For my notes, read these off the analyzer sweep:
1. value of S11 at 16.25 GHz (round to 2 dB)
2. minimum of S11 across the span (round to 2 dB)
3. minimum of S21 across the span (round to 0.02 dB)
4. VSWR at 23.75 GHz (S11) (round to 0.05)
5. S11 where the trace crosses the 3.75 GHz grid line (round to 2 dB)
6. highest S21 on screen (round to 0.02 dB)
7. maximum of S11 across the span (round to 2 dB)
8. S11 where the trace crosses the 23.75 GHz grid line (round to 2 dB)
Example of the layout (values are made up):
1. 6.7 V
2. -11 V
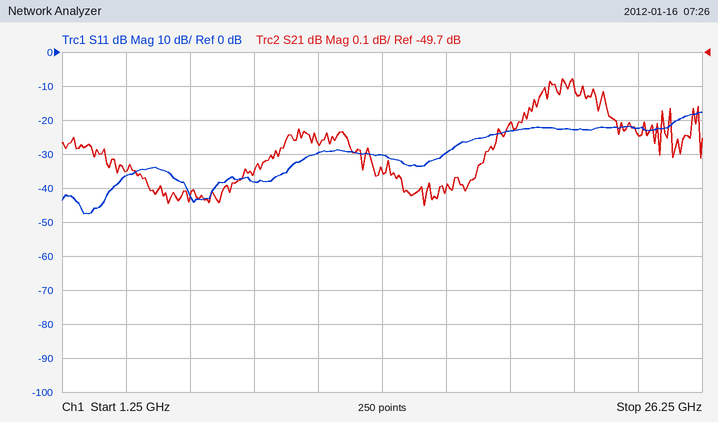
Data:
1. -30 dB
2. -48 dB
3. -50.16 dB
4. 1.15
5. -36 dB
6. -49.78 dB
7. -18 dB
8. -22 dB
